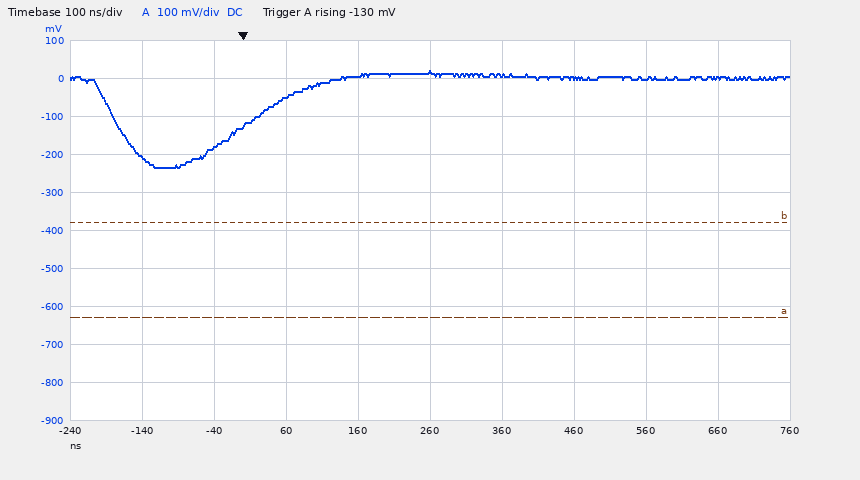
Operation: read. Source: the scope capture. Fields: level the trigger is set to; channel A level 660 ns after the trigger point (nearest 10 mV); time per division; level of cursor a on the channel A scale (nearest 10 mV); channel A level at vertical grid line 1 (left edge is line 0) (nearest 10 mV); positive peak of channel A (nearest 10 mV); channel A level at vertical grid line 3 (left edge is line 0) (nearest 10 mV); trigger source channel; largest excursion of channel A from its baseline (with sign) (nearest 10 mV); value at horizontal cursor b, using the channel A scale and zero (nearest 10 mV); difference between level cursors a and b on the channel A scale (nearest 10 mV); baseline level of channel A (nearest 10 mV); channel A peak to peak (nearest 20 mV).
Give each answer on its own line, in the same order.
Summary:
-130 mV
0 mV
100 ns
-630 mV
-210 mV
20 mV
-50 mV
channel A
-240 mV
-380 mV
250 mV
0 mV
260 mV
